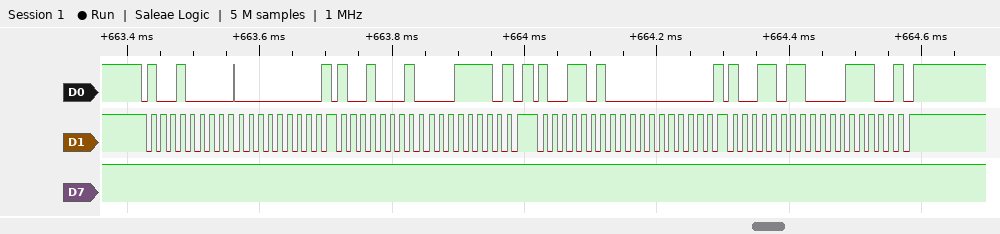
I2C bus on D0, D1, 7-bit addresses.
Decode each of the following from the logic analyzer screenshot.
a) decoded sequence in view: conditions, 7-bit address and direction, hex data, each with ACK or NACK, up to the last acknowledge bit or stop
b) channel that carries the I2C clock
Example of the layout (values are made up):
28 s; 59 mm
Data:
start, address 48 write ACK, 00 ACK, repeated start, address 48 read ACK, 1E NACK, stop, start, address 4D write ACK, 00 ACK, repeated start, address 4D read ACK, 1C NACK, stop; D1
